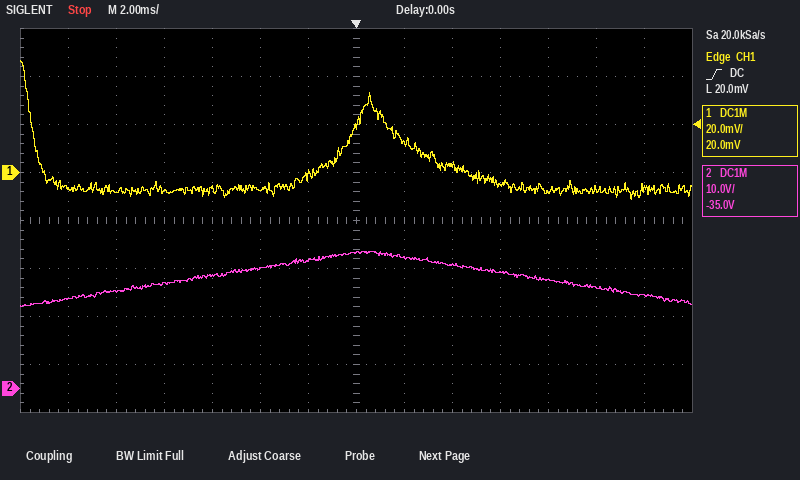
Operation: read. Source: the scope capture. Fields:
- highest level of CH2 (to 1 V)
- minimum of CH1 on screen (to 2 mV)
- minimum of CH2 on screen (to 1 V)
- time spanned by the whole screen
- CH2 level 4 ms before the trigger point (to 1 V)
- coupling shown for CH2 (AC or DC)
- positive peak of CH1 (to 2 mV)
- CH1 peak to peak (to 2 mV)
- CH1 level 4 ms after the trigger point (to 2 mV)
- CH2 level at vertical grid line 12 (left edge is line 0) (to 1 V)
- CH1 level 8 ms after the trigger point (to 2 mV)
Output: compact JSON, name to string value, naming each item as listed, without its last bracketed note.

{"highest level of CH2": "29 V", "minimum of CH1 on screen": "-12 mV", "minimum of CH2 on screen": "17 V", "time spanned by the whole screen": "28 ms", "CH2 level 4 ms before the trigger point": "25 V", "coupling shown for CH2": "DC", "positive peak of CH1": "46 mV", "CH1 peak to peak": "58 mV", "CH1 level 4 ms after the trigger point": "4 mV", "CH2 level at vertical grid line 12 (left edge is line 0)": "21 V", "CH1 level 8 ms after the trigger point": "-8 mV"}
